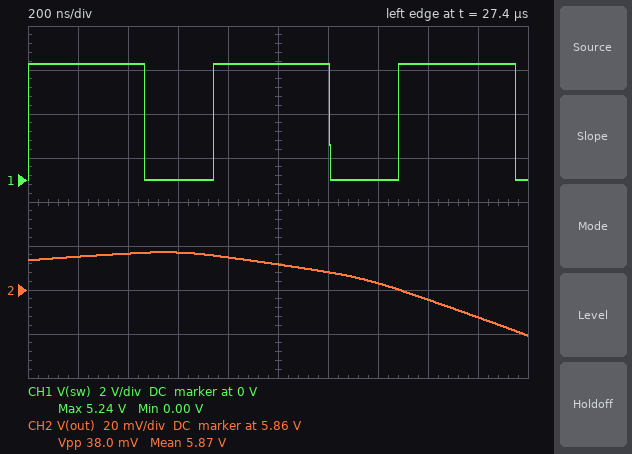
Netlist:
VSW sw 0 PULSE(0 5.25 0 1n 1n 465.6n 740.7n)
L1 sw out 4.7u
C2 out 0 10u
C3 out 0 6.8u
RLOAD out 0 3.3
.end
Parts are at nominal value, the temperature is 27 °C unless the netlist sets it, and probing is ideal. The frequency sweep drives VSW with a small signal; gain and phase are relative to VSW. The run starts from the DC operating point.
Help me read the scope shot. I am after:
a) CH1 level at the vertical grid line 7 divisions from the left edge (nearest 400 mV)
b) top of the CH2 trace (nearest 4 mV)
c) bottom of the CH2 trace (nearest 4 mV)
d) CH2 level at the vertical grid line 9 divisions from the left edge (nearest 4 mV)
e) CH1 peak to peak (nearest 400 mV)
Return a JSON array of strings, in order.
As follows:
["0 V", "5.876 V", "5.840 V", "5.848 V", "5.2 V"]
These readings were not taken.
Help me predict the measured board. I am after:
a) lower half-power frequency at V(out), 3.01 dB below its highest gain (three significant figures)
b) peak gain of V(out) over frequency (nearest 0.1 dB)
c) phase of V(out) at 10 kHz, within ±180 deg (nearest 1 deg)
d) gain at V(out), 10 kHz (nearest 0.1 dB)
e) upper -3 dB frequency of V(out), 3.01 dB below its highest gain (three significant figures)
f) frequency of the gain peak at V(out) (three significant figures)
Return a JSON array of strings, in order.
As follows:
["16.3 kHz", "15.9 dB", "-7 deg", "3.2 dB", "19.2 kHz", "17.8 kHz"]
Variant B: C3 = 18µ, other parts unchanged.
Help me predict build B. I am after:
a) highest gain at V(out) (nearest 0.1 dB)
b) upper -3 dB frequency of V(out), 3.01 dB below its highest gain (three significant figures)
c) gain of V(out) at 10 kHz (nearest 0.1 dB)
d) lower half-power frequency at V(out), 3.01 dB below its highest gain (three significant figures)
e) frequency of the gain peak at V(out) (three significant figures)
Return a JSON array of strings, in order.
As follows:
["18.1 dB", "14.7 kHz", "6.2 dB", "12.9 kHz", "13.8 kHz"]
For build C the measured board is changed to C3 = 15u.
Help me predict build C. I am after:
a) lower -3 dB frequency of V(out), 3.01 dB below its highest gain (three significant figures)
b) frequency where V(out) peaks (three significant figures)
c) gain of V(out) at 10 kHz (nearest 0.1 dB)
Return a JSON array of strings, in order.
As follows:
["13.6 kHz", "14.6 kHz", "5.3 dB"]
